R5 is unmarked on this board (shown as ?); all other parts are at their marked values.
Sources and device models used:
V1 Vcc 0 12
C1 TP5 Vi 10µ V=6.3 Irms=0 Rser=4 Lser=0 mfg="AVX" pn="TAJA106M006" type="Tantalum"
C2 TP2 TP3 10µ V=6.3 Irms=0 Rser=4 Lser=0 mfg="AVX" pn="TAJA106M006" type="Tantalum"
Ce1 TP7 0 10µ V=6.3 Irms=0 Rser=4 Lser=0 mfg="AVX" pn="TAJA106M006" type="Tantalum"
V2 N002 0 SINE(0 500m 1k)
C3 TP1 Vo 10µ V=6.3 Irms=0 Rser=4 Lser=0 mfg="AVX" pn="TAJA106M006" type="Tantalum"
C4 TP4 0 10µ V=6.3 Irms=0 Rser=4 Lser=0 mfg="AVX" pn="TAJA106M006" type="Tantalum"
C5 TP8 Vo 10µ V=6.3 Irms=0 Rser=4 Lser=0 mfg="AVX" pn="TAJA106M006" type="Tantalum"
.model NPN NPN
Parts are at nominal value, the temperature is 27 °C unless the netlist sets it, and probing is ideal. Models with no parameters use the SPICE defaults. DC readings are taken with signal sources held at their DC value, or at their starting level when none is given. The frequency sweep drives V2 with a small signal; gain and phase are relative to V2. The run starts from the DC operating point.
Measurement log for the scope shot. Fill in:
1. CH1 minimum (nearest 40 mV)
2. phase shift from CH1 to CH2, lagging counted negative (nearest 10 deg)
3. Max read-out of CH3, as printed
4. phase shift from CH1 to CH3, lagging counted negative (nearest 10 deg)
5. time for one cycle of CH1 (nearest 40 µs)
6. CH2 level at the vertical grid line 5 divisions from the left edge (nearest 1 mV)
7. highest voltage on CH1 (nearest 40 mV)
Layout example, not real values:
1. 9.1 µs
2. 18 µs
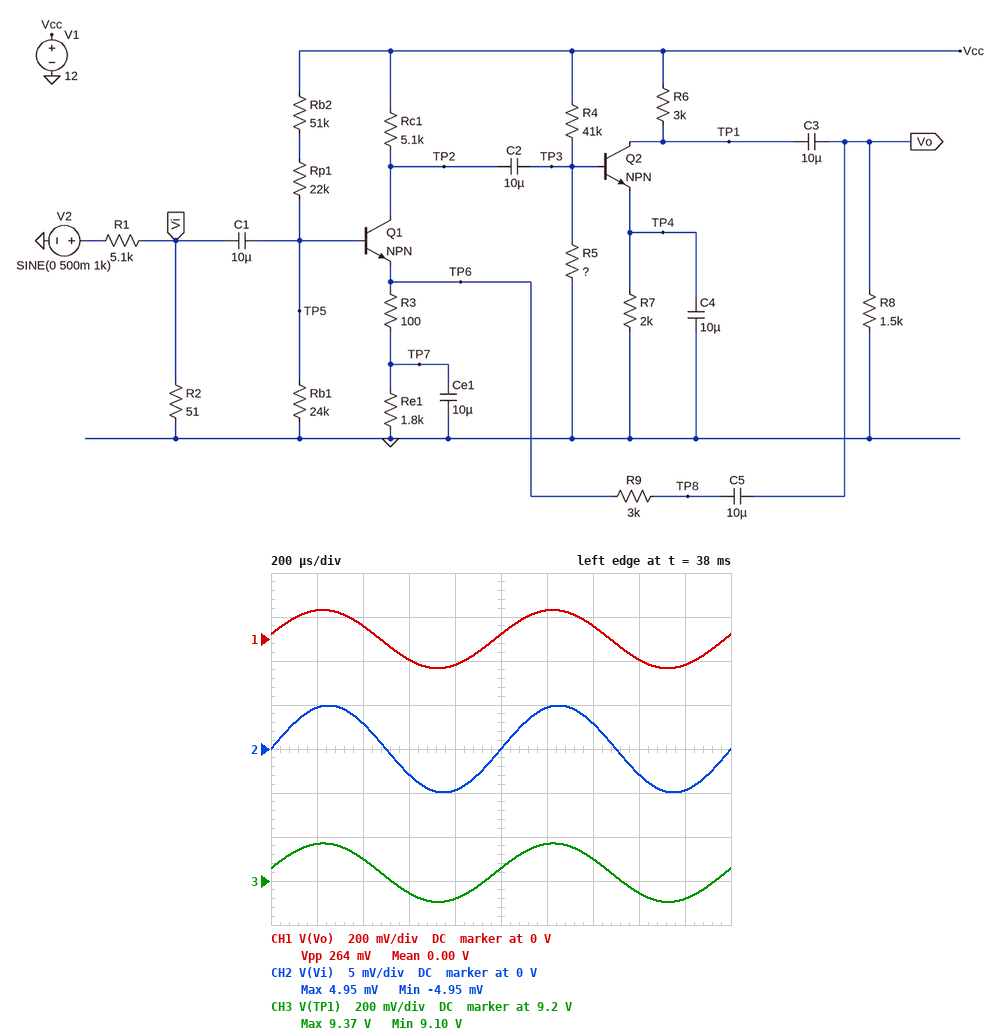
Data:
1. -120 mV
2. -10 deg
3. 9.37 V
4. 0 deg
5. 1.00 ms
6. 0 V
7. 120 mV
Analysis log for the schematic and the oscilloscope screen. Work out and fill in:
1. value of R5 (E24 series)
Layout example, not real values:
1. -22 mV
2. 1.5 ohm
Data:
1. 12 kΩ
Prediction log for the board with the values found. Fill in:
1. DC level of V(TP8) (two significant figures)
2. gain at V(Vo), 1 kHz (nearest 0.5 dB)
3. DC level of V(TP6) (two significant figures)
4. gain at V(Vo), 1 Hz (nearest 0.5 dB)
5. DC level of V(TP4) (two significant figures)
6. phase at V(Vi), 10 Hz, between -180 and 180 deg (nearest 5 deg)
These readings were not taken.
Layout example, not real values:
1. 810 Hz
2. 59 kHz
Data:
1. 2.0 V
2. -11.5 dB
3. 2.0 V
4. -57.0 dB
5. 1.9 V
6. 0 deg
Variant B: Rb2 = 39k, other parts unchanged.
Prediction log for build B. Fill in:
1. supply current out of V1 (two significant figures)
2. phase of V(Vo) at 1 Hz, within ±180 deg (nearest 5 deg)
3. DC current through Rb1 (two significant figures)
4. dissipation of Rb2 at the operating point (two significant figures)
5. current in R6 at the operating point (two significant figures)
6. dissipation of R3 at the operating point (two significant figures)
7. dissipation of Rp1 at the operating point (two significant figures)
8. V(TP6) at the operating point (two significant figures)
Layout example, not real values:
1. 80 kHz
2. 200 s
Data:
1. 2.5 mA
2. 160 deg
3. 130 µA
4. 820 µW
5. 920 µA
6. 160 µW
7. 460 µW
8. 2.4 V
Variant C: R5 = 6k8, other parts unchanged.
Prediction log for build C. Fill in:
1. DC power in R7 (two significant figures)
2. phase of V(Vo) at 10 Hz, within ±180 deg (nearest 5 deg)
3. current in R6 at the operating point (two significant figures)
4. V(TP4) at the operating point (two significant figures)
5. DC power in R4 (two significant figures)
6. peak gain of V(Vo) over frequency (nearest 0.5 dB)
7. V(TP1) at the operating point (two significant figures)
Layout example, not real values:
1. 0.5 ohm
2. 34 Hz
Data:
1. 430 µW
2. 85 deg
3. 460 µA
4. 930 mV
5. 2.6 mW
6. -12.0 dB
7. 11 V
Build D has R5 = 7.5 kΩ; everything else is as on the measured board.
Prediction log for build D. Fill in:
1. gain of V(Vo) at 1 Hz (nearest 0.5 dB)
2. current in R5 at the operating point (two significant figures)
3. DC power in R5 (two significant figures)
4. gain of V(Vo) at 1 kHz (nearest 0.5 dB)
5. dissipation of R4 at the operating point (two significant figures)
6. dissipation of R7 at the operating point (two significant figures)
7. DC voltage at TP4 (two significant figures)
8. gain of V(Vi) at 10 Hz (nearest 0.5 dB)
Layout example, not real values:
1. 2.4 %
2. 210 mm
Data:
1. -59.0 dB
2. 240 µA
3. 440 µW
4. -12.0 dB
5. 2.5 mW
6. 570 µW
7. 1.1 V
8. -40.0 dB
